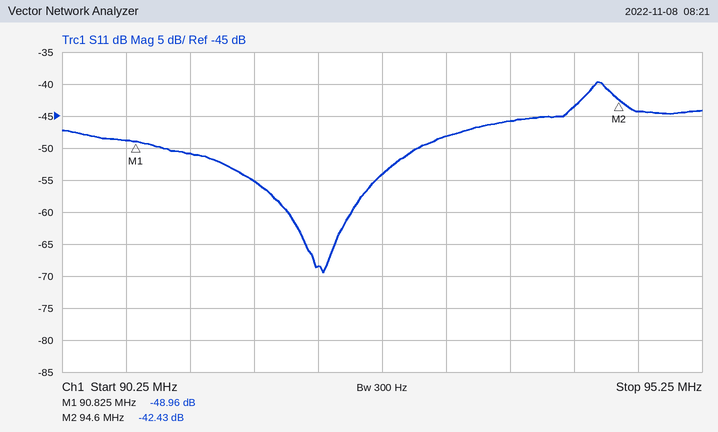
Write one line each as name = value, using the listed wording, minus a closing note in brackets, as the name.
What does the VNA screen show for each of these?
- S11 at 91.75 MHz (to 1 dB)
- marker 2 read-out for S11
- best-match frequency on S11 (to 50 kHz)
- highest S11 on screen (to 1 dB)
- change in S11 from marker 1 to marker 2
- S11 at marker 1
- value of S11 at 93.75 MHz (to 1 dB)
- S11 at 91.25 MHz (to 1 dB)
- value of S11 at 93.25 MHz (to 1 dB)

S11 at 91.75 MHz = -55 dB
marker 2 read-out for S11 = -42.43 dB
best-match frequency on S11 = 92.30 MHz
highest S11 on screen = -40 dB
change in S11 from marker 1 to marker 2 = 6.53 dB
S11 at marker 1 = -48.96 dB
value of S11 at 93.75 MHz = -46 dB
S11 at 91.25 MHz = -51 dB
value of S11 at 93.25 MHz = -48 dB
